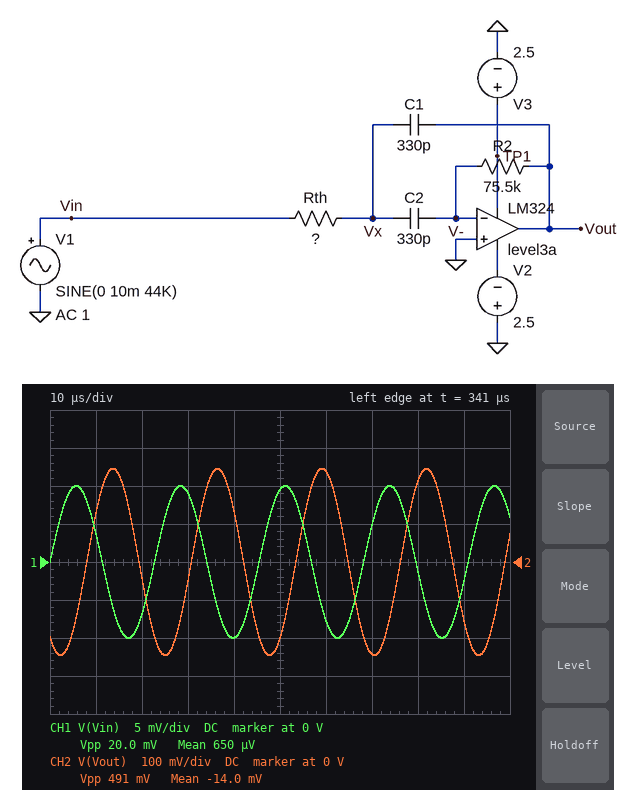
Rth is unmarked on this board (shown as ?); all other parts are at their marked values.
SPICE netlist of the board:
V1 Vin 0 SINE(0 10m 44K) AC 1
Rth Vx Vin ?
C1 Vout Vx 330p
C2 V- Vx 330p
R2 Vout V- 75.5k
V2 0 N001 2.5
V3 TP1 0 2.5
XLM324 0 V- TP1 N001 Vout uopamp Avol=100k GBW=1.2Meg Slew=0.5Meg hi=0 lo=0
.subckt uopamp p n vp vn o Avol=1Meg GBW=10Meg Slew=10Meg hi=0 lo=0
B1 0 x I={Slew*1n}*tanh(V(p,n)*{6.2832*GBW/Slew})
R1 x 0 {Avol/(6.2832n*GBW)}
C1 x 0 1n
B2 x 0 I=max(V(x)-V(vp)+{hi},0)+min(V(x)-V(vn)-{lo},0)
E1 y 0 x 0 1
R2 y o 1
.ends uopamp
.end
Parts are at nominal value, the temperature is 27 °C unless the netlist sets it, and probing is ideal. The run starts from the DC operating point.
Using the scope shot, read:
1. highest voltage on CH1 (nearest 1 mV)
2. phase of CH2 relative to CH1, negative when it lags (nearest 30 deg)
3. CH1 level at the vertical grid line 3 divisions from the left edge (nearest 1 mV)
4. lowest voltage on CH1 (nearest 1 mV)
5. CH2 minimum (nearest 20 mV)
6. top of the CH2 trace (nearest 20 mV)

10 mV
-120 deg
9 mV
-10 mV
-240 mV
240 mV
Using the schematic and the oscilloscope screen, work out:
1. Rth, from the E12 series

820 Ω
